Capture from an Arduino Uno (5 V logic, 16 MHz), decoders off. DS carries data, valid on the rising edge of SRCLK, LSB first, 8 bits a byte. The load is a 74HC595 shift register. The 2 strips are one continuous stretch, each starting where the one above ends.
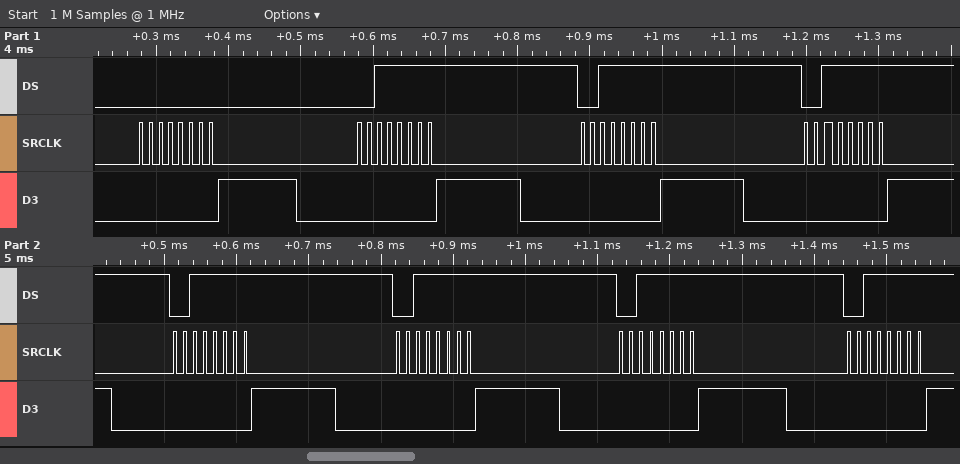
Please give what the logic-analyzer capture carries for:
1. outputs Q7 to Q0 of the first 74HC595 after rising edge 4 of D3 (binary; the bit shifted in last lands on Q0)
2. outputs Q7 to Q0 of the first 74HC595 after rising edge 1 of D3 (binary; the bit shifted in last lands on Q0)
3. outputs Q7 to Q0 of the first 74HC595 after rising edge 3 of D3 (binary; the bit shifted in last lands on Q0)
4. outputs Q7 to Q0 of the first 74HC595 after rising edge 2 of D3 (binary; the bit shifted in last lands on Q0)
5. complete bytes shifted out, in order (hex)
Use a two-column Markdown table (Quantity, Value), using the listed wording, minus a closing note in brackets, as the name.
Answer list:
| Quantity | Value |
|---|---|
| outputs Q7 to Q0 of the first 74HC595 after rising edge 4 of D3 | 00111111 |
| outputs Q7 to Q0 of the first 74HC595 after rising edge 1 of D3 | 00000000 |
| outputs Q7 to Q0 of the first 74HC595 after rising edge 3 of D3 | 00111111 |
| outputs Q7 to Q0 of the first 74HC595 after rising edge 2 of D3 | 00111111 |
| complete bytes shifted out, in order | 0x00 0xFC 0xFC 0xFC 0xFC 0xFC 0xFC 0xFC |
